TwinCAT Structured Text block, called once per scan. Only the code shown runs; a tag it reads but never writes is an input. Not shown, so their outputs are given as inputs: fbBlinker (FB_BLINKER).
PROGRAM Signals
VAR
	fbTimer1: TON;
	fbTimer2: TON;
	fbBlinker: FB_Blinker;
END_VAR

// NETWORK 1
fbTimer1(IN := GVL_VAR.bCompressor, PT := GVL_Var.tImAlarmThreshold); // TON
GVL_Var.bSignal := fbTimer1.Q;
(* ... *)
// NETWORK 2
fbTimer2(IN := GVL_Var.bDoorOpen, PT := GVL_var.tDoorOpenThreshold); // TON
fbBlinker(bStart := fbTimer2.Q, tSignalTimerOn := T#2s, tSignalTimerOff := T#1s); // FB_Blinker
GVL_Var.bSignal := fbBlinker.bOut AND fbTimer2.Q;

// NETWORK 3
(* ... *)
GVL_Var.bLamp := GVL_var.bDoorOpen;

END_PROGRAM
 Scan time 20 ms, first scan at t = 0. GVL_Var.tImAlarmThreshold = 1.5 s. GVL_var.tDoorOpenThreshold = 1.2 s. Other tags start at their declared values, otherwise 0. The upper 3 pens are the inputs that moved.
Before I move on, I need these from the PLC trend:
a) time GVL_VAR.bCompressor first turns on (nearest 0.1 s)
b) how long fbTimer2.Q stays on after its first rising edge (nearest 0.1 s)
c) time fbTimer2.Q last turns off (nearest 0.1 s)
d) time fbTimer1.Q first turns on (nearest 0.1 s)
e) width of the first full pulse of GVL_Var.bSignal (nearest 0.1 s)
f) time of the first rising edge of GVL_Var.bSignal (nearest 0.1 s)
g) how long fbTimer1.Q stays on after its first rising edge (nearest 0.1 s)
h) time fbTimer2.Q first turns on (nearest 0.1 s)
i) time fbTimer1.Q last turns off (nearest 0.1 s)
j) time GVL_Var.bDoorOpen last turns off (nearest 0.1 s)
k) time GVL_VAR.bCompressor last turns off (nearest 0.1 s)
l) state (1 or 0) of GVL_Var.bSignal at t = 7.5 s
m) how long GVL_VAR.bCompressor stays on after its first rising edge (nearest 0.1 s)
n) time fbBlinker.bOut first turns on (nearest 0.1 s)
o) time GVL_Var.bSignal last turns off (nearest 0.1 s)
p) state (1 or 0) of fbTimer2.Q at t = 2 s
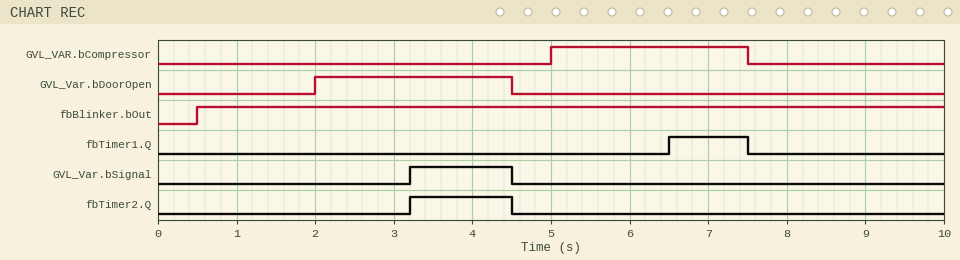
5.0 s
1.3 s
4.5 s
6.5 s
1.3 s
3.2 s
1.0 s
3.2 s
7.5 s
4.5 s
7.5 s
0
2.5 s
0.5 s
4.5 s
0
